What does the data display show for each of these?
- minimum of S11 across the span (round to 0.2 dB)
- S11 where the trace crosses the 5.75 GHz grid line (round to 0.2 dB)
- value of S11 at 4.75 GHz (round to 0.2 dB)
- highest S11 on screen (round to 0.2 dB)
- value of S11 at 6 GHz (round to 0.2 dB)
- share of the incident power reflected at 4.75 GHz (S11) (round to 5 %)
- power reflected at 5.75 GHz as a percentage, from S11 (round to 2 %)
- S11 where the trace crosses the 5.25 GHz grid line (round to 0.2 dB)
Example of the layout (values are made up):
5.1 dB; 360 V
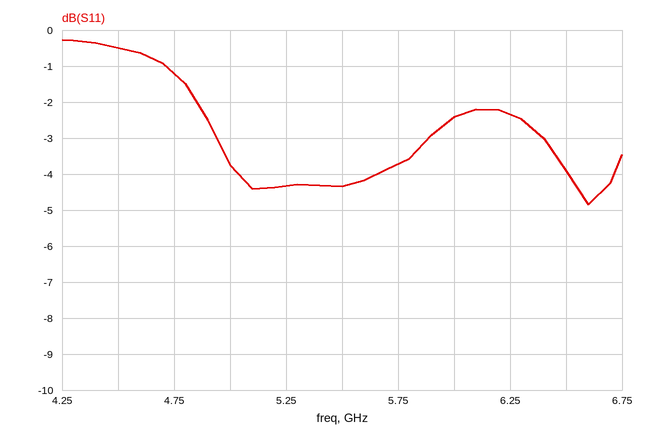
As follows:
-4.8 dB; -3.8 dB; -1.2 dB; -0.2 dB; -2.4 dB; 75 %; 42 %; -4.4 dB
